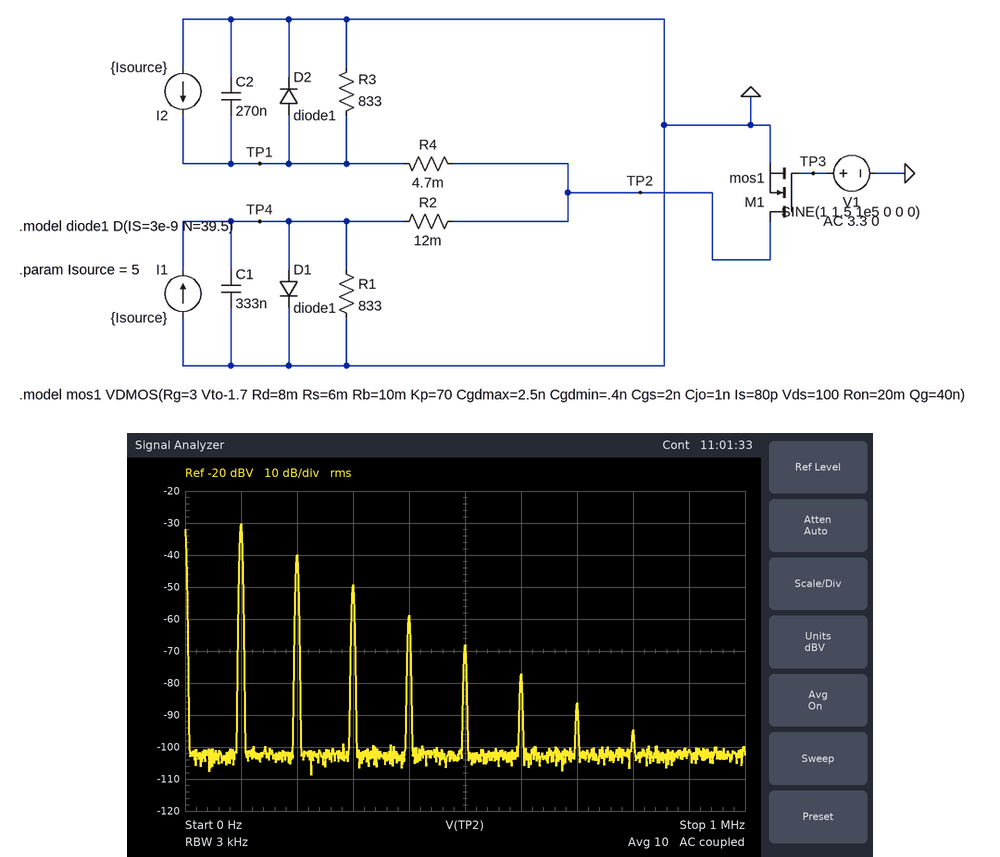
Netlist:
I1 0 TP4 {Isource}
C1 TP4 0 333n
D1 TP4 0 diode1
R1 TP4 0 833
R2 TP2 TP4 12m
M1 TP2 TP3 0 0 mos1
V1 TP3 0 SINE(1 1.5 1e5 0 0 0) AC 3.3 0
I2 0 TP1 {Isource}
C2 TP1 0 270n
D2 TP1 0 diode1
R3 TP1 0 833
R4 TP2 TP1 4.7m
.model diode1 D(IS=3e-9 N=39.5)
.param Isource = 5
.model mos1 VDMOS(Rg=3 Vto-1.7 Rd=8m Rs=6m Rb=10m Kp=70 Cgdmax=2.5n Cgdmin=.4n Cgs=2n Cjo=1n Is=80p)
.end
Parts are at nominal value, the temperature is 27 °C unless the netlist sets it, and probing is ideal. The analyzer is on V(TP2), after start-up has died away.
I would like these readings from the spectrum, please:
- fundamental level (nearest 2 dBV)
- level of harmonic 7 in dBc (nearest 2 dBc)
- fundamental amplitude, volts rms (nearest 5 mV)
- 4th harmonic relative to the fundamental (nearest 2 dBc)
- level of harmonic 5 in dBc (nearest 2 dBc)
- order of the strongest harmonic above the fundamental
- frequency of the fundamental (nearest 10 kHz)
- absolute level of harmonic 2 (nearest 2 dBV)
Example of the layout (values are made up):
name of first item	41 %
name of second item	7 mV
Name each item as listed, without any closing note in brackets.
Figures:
fundamental level	-30 dBV
level of harmonic 7 in dBc	-56 dBc
fundamental amplitude, volts rms	30 mV
4th harmonic relative to the fundamental	-28 dBc
level of harmonic 5 in dBc	-38 dBc
order of the strongest harmonic above the fundamental	2
frequency of the fundamental	100 kHz
absolute level of harmonic 2	-40 dBV
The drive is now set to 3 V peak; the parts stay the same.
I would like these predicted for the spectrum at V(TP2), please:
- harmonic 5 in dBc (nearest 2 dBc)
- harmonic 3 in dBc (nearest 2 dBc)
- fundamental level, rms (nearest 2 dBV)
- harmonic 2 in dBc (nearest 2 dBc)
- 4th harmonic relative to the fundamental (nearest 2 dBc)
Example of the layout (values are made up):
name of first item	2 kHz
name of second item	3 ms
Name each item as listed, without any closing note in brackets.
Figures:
harmonic 5 in dBc	-22 dBc
harmonic 3 in dBc	-8 dBc
fundamental level, rms	16 dBV
harmonic 2 in dBc	-2 dBc
4th harmonic relative to the fundamental	-16 dBc
